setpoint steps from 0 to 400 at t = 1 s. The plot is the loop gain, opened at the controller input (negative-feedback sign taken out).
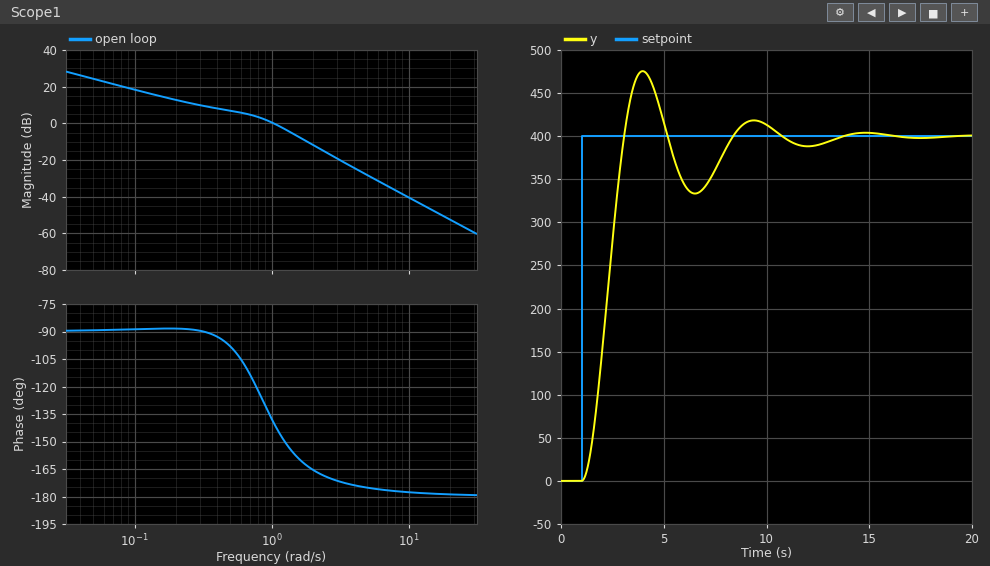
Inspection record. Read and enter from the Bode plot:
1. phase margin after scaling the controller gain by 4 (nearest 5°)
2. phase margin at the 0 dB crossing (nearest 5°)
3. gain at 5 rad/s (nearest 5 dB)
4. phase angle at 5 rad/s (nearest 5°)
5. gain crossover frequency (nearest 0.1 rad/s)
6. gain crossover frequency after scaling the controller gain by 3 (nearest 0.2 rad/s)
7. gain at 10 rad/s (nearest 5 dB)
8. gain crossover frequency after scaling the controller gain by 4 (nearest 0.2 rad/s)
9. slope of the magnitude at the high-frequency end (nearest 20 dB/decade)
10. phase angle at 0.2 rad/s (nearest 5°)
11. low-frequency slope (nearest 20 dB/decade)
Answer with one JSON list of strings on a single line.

["15°", "40°", "-30 dB", "-175°", "1.0 rad/s", "1.8 rad/s", "-40 dB", "2.0 rad/s", "-40 dB/decade", "-90°", "-20 dB/decade"]
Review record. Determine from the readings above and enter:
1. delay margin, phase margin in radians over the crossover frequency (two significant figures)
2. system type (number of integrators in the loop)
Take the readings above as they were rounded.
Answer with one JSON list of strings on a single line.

["0.70 s", "1"]
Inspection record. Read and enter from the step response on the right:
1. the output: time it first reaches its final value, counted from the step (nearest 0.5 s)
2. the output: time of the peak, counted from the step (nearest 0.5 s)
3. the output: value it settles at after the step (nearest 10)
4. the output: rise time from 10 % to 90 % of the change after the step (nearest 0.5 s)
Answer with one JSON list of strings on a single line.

["2.0 s", "3.0 s", "400", "1.5 s"]
